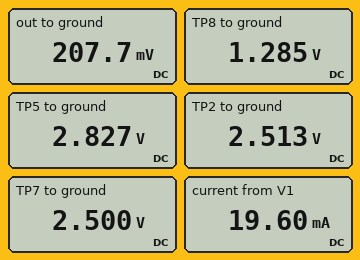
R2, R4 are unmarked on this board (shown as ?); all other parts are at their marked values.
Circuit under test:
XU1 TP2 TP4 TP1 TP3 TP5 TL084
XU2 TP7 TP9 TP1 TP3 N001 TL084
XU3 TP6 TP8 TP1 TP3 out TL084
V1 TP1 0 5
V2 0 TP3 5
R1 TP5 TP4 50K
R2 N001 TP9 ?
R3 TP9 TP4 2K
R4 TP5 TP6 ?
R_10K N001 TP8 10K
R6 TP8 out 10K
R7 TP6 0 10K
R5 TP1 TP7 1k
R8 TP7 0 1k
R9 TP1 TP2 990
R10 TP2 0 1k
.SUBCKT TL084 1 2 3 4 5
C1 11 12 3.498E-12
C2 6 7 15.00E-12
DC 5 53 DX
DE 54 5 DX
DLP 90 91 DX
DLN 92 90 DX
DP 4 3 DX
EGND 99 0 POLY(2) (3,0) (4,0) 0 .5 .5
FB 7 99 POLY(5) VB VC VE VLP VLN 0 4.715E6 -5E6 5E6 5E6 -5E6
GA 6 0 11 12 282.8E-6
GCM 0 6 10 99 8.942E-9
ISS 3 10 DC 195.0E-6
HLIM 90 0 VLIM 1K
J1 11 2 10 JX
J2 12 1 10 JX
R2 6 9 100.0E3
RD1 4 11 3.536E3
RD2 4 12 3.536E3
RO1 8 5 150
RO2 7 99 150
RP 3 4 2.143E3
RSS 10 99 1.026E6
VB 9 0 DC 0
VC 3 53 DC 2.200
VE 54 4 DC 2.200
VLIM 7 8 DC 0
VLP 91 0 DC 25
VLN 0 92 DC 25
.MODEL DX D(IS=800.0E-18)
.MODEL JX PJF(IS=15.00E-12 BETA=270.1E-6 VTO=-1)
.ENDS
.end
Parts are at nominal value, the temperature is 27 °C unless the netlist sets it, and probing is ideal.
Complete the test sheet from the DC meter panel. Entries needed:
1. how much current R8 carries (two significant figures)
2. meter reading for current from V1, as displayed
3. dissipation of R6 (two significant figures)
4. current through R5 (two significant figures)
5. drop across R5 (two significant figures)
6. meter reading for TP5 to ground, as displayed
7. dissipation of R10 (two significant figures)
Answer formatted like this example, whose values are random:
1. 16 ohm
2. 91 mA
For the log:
1. 2.5 mA
2. 19.60 mA
3. 120 µW
4. 2.5 mA
5. 2.5 V
6. 2.827 V
7. 6.3 mW
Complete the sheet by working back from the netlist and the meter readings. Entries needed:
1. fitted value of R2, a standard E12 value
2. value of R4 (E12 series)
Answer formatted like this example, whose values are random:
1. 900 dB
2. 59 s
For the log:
1. 22 kΩ
2. 12 kΩ
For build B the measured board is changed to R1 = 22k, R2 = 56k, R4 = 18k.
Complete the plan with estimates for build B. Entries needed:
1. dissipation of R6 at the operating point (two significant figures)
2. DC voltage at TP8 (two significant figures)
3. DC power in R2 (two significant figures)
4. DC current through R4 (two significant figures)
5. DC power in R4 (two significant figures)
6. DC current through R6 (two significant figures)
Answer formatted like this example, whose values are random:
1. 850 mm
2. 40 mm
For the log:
1. 140 µW
2. 950 mV
3. 2.2 µW
4. 95 µA
5. 160 µW
6. 120 µA
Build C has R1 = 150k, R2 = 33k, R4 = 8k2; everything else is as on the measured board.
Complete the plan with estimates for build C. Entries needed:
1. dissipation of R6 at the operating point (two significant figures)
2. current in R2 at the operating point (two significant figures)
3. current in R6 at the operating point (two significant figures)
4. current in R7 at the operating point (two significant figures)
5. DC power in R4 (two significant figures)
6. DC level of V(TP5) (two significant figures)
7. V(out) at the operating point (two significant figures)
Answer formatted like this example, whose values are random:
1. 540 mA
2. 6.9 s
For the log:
1. 24 µW
2. 5.4 µA
3. 49 µA
4. 180 µA
5. 270 µW
6. 3.3 V
7. 1.3 V
